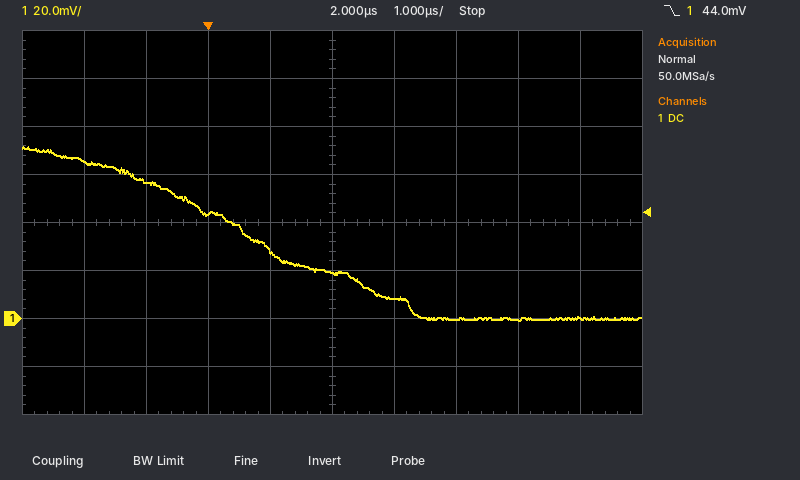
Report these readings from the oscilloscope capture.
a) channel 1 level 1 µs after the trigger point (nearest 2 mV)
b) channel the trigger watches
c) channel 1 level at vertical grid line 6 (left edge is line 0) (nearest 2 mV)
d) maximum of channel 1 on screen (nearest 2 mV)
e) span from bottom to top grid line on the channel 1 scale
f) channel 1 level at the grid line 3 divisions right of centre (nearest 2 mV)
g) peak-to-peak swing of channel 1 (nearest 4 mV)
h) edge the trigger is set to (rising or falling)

28 mV
channel 1
8 mV
72 mV
160 mV
0 mV
72 mV
falling
